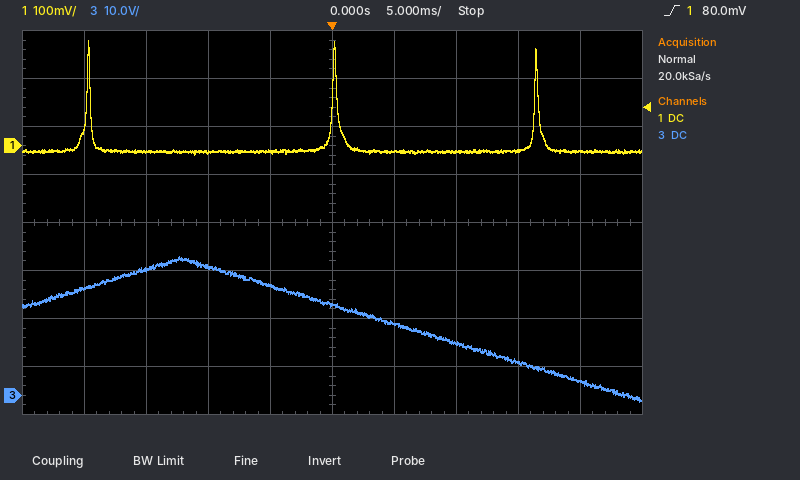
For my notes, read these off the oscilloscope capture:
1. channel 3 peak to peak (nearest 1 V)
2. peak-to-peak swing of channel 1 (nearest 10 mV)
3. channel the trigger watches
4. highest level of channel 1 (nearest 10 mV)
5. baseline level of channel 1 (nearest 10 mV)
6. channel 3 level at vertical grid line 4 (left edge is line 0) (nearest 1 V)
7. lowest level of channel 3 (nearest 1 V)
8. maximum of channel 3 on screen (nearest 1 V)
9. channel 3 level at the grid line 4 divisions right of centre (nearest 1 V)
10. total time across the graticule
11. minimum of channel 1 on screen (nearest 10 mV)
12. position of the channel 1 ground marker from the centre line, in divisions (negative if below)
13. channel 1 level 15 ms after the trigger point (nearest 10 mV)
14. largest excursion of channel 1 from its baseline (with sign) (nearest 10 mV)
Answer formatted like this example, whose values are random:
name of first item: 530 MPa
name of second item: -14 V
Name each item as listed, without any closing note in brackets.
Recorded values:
channel 3 peak to peak: 30 V
peak-to-peak swing of channel 1: 240 mV
channel the trigger watches: channel 1
highest level of channel 1: 220 mV
baseline level of channel 1: -10 mV
channel 3 level at vertical grid line 4 (left edge is line 0): 23 V
lowest level of channel 3: -1 V
maximum of channel 3 on screen: 29 V
channel 3 level at the grid line 4 divisions right of centre: 3 V
total time across the graticule: 50 ms
minimum of channel 1 on screen: -20 mV
position of the channel 1 ground marker from the centre line, in divisions: +1.6 div
channel 1 level 15 ms after the trigger point: -10 mV
largest excursion of channel 1 from its baseline (with sign): +230 mV
